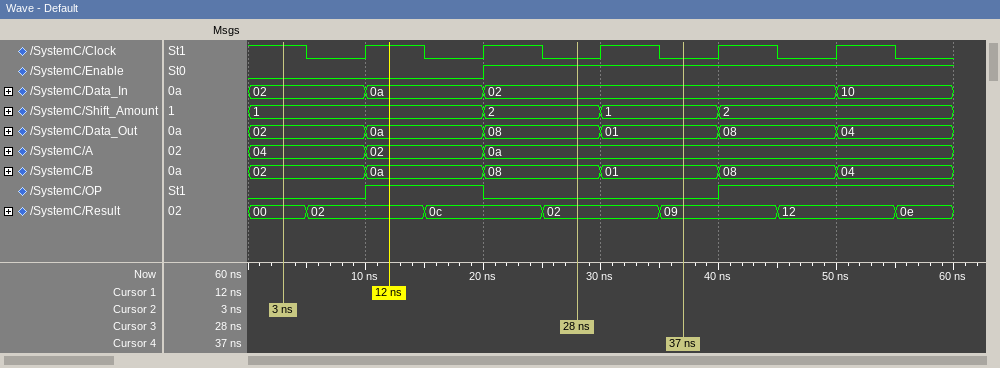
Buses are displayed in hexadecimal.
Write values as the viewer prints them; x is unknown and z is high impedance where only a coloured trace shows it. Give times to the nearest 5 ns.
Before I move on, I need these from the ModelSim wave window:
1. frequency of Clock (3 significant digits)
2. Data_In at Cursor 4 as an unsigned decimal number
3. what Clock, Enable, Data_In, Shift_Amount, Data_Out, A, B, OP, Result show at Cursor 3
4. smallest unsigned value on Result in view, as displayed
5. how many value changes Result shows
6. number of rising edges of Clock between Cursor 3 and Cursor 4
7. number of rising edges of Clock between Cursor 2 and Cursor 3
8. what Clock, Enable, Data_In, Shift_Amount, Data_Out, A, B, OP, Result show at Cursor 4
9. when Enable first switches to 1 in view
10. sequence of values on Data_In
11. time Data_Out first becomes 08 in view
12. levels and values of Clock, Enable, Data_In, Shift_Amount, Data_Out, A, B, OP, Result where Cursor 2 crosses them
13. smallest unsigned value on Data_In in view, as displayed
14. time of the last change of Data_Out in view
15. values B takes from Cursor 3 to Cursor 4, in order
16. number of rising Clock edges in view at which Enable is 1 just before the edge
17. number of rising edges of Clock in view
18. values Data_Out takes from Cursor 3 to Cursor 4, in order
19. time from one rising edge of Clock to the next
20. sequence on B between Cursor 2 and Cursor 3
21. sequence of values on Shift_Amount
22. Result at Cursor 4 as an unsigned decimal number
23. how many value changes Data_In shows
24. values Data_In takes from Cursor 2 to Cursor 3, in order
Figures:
100 MHz
2
Clock=0, Enable=1, Data_In=02, Shift_Amount=2, Data_Out=08, A=0a, B=08, OP=0, Result=02
00
6
1
2
Clock=0, Enable=1, Data_In=02, Shift_Amount=1, Data_Out=01, A=0a, B=01, OP=0, Result=09
20 ns
02, 0a, 02, 10
20 ns
Clock=1, Enable=0, Data_In=02, Shift_Amount=1, Data_Out=02, A=04, B=02, OP=0, Result=00
02
50 ns
08, 01
3
5
08, 01
10 ns
02, 0a, 08
1, 2, 1, 2
9
3
02, 0a, 02
